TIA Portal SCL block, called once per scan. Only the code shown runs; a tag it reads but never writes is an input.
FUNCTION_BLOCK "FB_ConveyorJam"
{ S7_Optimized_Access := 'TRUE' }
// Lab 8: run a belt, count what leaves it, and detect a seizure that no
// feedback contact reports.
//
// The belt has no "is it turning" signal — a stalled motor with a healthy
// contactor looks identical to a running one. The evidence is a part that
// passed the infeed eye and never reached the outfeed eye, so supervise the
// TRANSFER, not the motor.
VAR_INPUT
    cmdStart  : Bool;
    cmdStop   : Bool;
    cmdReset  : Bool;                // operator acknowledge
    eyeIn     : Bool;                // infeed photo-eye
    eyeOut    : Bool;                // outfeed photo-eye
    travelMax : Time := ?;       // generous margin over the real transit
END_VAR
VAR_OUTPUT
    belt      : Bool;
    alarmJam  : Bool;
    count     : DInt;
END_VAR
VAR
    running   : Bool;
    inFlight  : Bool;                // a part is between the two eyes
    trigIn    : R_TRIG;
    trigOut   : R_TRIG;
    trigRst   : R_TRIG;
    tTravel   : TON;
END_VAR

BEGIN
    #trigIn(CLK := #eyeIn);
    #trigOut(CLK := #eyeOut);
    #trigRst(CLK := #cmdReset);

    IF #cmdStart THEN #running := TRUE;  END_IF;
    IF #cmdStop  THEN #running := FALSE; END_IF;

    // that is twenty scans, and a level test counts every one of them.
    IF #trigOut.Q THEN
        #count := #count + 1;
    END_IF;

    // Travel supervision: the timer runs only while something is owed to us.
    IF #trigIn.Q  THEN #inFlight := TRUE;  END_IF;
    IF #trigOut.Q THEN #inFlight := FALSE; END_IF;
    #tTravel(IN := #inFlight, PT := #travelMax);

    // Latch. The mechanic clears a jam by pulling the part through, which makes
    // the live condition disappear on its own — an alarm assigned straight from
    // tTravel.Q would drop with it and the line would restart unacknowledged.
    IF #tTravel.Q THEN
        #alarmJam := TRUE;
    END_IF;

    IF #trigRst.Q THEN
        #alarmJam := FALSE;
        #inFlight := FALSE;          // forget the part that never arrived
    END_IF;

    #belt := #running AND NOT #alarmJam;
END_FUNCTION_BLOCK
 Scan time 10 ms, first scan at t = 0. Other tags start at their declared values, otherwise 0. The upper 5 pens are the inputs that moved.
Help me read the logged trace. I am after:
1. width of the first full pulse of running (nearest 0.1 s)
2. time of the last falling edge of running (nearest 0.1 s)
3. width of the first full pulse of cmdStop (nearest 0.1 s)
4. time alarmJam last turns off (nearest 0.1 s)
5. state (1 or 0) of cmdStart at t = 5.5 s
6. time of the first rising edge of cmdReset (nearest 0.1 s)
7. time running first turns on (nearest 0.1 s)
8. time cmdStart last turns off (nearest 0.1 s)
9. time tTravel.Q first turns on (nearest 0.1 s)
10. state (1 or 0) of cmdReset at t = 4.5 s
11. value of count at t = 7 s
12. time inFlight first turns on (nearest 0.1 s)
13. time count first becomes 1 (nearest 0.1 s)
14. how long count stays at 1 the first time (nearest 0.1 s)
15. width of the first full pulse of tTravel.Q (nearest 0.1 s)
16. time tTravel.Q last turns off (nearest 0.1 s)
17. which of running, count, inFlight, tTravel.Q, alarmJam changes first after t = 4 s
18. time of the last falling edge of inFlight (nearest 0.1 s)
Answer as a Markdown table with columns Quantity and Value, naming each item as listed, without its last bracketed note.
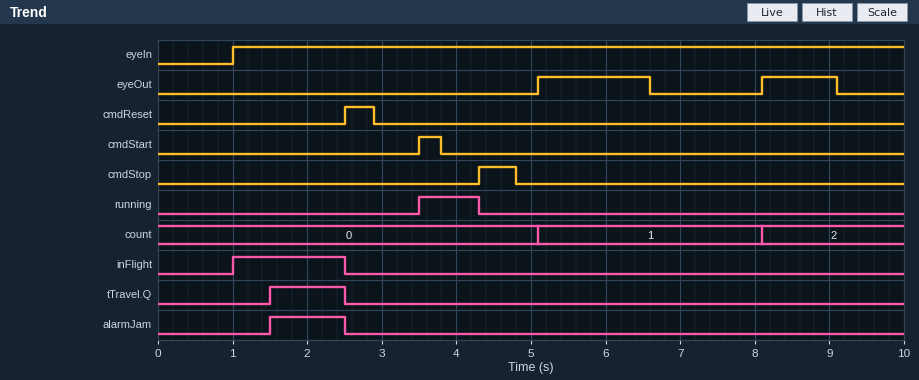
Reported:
| Quantity | Value |
|---|---|
| width of the first full pulse of running | 0.8 s |
| time of the last falling edge of running | 4.3 s |
| width of the first full pulse of cmdStop | 0.5 s |
| time alarmJam last turns off | 2.5 s |
| state (1 or 0) of cmdStart at t = 5.5 s | 0 |
| time of the first rising edge of cmdReset | 2.5 s |
| time running first turns on | 3.5 s |
| time cmdStart last turns off | 3.8 s |
| time tTravel.Q first turns on | 1.5 s |
| state (1 or 0) of cmdReset at t = 4.5 s | 0 |
| value of count at t = 7 s | 1 |
| time inFlight first turns on | 1.0 s |
| time count first becomes 1 | 5.1 s |
| how long count stays at 1 the first time | 3.0 s |
| width of the first full pulse of tTravel.Q | 1.0 s |
| time tTravel.Q last turns off | 2.5 s |
| which of running, count, inFlight, tTravel.Q, alarmJam changes first after t = 4 s | running |
| time of the last falling edge of inFlight | 2.5 s |
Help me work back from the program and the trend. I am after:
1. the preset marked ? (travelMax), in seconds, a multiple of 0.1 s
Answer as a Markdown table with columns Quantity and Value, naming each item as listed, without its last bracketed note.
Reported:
| Quantity | Value |
|---|---|
| the preset marked ? (travelMax), in seconds, a multiple of 0.1 s | 0.5 s |
